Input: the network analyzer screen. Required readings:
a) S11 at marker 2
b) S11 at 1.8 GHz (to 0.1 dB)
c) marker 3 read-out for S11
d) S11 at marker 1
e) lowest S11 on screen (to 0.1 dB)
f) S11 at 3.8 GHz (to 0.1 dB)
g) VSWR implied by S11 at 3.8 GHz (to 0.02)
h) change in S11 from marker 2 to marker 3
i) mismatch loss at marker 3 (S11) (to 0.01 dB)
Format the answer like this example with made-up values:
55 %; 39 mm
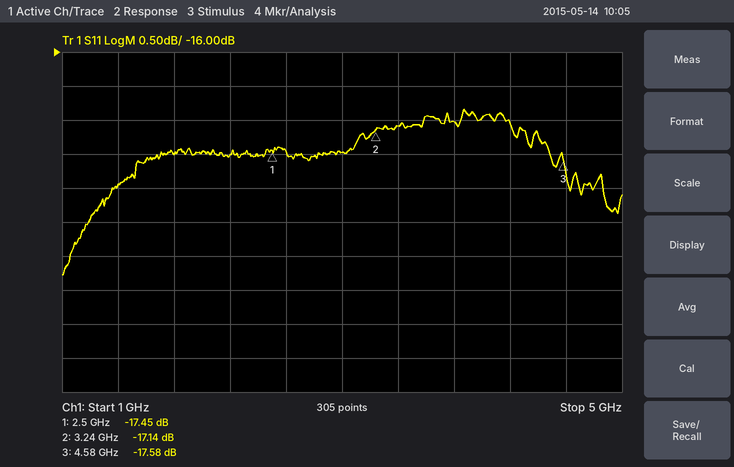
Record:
-17.14 dB; -17.5 dB; -17.58 dB; -17.45 dB; -19.3 dB; -17.0 dB; 1.32; -0.44 dB; 0.08 dB
